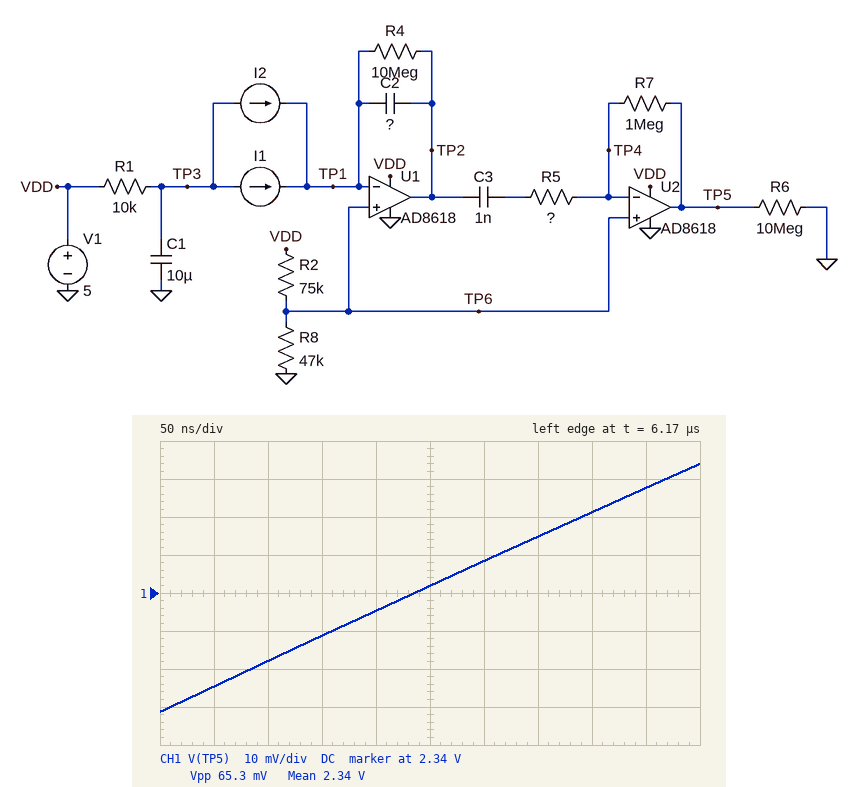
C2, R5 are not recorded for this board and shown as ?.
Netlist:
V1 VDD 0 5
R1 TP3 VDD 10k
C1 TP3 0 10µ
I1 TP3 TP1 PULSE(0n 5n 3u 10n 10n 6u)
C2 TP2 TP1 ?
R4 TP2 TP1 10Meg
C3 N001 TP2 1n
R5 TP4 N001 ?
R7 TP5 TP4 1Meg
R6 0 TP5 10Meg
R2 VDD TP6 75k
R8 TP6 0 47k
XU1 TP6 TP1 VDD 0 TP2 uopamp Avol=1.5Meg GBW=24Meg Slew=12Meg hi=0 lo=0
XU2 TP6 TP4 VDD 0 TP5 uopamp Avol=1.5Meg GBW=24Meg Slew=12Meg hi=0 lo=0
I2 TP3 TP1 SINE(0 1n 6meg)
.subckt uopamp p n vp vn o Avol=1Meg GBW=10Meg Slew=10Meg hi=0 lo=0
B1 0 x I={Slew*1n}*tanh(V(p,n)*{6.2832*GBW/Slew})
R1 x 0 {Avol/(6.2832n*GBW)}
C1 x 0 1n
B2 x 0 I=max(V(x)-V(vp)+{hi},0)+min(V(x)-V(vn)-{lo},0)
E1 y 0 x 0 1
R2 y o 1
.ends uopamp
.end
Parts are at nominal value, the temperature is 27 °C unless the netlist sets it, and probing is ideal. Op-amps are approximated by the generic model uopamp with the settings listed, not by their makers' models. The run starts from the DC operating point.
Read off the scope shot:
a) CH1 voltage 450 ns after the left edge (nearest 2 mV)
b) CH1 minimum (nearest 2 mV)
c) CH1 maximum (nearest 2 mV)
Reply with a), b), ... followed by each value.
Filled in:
a) 2.368 V
b) 2.308 V
c) 2.374 V
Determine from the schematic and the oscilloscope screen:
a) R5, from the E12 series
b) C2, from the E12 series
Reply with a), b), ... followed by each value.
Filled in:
a) 8.2 kΩ
b) 3.3 pF
